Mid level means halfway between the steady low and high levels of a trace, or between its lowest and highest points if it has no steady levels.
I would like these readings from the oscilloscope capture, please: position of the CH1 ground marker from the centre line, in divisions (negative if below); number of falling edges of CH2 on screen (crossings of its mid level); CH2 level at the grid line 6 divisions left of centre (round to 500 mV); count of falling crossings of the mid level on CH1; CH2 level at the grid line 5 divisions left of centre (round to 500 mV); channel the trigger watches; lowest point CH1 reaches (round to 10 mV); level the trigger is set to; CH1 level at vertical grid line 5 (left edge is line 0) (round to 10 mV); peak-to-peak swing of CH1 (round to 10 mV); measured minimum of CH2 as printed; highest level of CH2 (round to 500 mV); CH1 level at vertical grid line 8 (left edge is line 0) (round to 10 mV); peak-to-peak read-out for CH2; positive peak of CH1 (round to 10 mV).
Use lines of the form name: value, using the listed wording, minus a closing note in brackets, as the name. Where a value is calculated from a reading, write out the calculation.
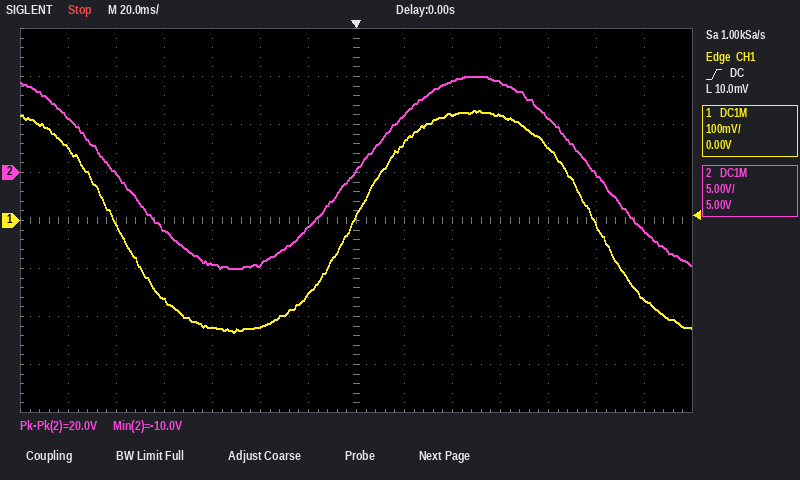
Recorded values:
position of the CH1 ground marker from the centre line, in divisions: 0.0 div
number of falling edges of CH2 on screen: 2
CH2 level at the grid line 6 divisions left of centre: 5.5 V
count of falling crossings of the mid level on CH1: 2
CH2 level at the grid line 5 divisions left of centre: 0.0 V
channel the trigger watches: CH1
lowest point CH1 reaches: -230 mV
level the trigger is set to: 10.0 mV
CH1 level at vertical grid line 5 (left edge is line 0): -220 mV
peak-to-peak swing of CH1: 230 mV − (-230 mV) = 460 mV
measured minimum of CH2 as printed: -10.0 V
highest level of CH2: 10.0 V
CH1 level at vertical grid line 8 (left edge is line 0): 160 mV
peak-to-peak read-out for CH2: 20.0 V
positive peak of CH1: 230 mV
